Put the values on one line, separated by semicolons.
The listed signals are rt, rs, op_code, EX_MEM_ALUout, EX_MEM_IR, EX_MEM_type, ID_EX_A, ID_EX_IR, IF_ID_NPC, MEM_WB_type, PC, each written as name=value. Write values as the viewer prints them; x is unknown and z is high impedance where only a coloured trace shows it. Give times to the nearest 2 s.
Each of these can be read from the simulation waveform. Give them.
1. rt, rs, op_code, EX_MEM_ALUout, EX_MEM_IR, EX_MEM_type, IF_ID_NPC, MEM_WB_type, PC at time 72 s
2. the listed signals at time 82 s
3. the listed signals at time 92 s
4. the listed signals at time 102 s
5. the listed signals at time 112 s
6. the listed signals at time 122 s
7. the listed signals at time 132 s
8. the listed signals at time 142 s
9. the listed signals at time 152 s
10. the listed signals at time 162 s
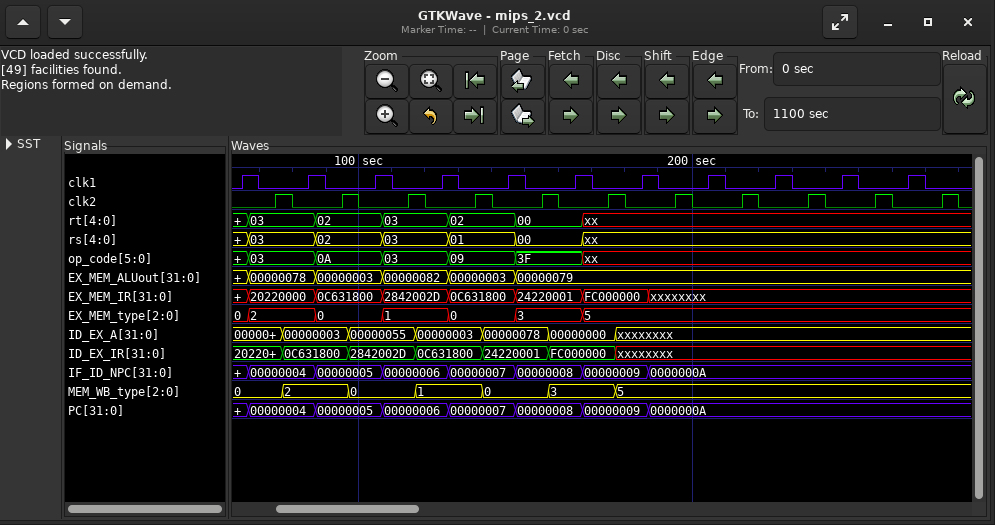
rt=03, rs=03, op_code=03, EX_MEM_ALUout=00000078, EX_MEM_IR=20220000, EX_MEM_type=2, IF_ID_NPC=00000004, MEM_WB_type=0, PC=00000004; rt=03, rs=03, op_code=03, EX_MEM_ALUout=00000078, EX_MEM_IR=20220000, EX_MEM_type=2, ID_EX_A=00000003, ID_EX_IR=0C631800, IF_ID_NPC=00000004, MEM_WB_type=2, PC=00000004; rt=02, rs=02, op_code=0A, EX_MEM_ALUout=00000003, EX_MEM_IR=0C631800, EX_MEM_type=0, ID_EX_A=00000003, ID_EX_IR=0C631800, IF_ID_NPC=00000005, MEM_WB_type=2, PC=00000005; rt=02, rs=02, op_code=0A, EX_MEM_ALUout=00000003, EX_MEM_IR=0C631800, EX_MEM_type=0, ID_EX_A=00000055, ID_EX_IR=2842002D, IF_ID_NPC=00000005, MEM_WB_type=0, PC=00000005; rt=03, rs=03, op_code=03, EX_MEM_ALUout=00000082, EX_MEM_IR=2842002D, EX_MEM_type=1, ID_EX_A=00000055, ID_EX_IR=2842002D, IF_ID_NPC=00000006, MEM_WB_type=0, PC=00000006; rt=03, rs=03, op_code=03, EX_MEM_ALUout=00000082, EX_MEM_IR=2842002D, EX_MEM_type=1, ID_EX_A=00000003, ID_EX_IR=0C631800, IF_ID_NPC=00000006, MEM_WB_type=1, PC=00000006; rt=02, rs=01, op_code=09, EX_MEM_ALUout=00000003, EX_MEM_IR=0C631800, EX_MEM_type=0, ID_EX_A=00000003, ID_EX_IR=0C631800, IF_ID_NPC=00000007, MEM_WB_type=1, PC=00000007; rt=02, rs=01, op_code=09, EX_MEM_ALUout=00000003, EX_MEM_IR=0C631800, EX_MEM_type=0, ID_EX_A=00000078, ID_EX_IR=24220001, IF_ID_NPC=00000007, MEM_WB_type=0, PC=00000007; rt=00, rs=00, op_code=3F, EX_MEM_ALUout=00000079, EX_MEM_IR=24220001, EX_MEM_type=3, ID_EX_A=00000078, ID_EX_IR=24220001, IF_ID_NPC=00000008, MEM_WB_type=0, PC=00000008; rt=00, rs=00, op_code=3F, EX_MEM_ALUout=00000079, EX_MEM_IR=24220001, EX_MEM_type=3, ID_EX_A=00000000, ID_EX_IR=FC000000, IF_ID_NPC=00000008, MEM_WB_type=3, PC=00000008
